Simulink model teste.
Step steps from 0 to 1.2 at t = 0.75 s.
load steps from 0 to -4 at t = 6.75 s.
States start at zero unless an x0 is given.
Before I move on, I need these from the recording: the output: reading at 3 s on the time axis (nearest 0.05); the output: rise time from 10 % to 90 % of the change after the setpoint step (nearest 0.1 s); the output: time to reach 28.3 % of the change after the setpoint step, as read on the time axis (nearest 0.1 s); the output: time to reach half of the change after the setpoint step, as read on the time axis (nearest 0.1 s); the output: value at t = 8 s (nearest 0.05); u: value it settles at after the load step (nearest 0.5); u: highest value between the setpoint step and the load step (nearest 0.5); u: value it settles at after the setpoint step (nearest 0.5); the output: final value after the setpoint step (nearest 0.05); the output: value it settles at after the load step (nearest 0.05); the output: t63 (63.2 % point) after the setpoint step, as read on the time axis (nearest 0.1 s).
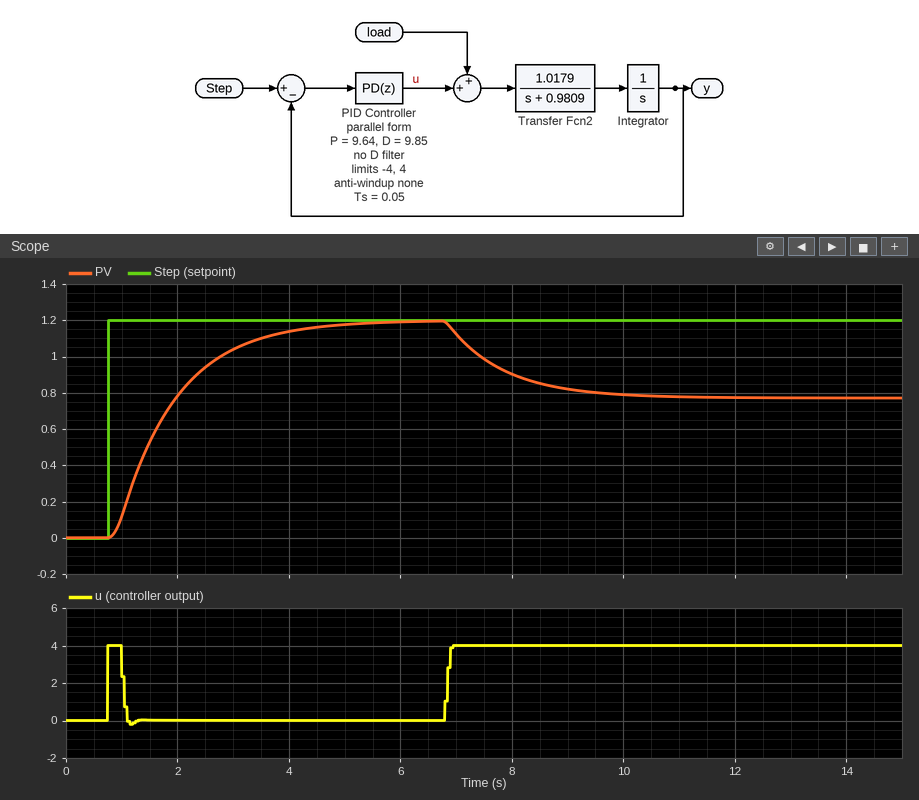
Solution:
1.05
2.3 s
1.2 s
1.6 s
0.90
4.0
4.0
0.0
1.20
0.75
1.9 s
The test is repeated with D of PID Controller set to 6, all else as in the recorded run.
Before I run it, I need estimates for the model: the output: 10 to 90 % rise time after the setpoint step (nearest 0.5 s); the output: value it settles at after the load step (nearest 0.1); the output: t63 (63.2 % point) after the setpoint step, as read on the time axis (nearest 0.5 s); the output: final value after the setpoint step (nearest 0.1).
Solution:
1.5 s
0.6
1.5 s
1.2
